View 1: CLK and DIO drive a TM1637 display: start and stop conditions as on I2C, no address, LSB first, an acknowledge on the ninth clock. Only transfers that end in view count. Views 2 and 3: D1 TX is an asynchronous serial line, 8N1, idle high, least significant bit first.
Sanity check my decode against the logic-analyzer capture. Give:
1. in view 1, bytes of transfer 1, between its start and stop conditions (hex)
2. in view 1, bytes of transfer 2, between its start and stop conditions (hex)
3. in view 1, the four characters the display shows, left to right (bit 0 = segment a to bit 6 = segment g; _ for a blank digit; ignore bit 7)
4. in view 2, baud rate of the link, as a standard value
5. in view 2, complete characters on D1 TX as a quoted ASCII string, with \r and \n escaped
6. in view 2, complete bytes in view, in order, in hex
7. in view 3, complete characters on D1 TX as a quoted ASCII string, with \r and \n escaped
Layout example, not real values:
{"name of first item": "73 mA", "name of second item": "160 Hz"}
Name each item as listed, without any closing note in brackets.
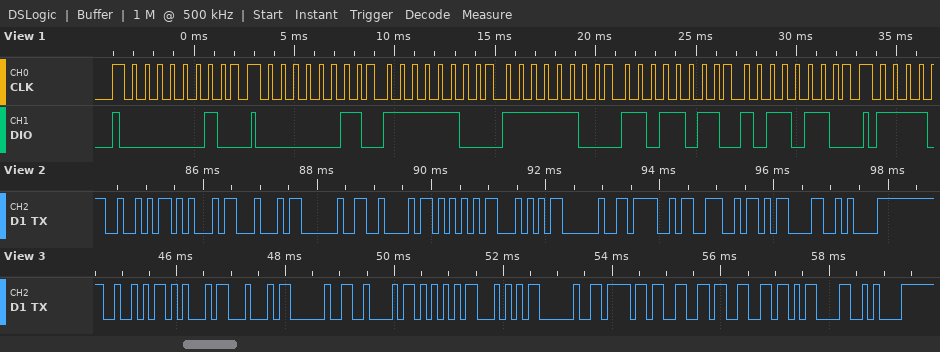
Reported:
{"in view 1, bytes of transfer 1, between its start and stop conditions": "40", "in view 1, bytes of transfer 2, between its start and stop conditions": "C0 3F 3F DB 6D", "in view 1, the four characters the display shows, left to right": "0025", "in view 2, baud rate of the link, as a standard value": "9600 baud", "in view 2, complete characters on D1 TX as a quoted ASCII string, with \\r and \\n escaped": "\"RED BUT ON\\r\\n\"", "in view 2, complete bytes in view, in order, in hex": "0x52 0x45 0x44 0x20 0x42 0x55 0x54 0x20 0x4F 0x4E 0x0D 0x0A", "in view 3, complete characters on D1 TX as a quoted ASCII string, with \\r and \\n escaped": "\"RED BUT off\\r\\n\""}
